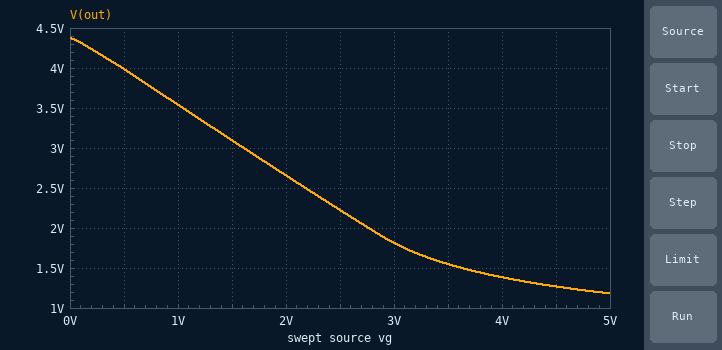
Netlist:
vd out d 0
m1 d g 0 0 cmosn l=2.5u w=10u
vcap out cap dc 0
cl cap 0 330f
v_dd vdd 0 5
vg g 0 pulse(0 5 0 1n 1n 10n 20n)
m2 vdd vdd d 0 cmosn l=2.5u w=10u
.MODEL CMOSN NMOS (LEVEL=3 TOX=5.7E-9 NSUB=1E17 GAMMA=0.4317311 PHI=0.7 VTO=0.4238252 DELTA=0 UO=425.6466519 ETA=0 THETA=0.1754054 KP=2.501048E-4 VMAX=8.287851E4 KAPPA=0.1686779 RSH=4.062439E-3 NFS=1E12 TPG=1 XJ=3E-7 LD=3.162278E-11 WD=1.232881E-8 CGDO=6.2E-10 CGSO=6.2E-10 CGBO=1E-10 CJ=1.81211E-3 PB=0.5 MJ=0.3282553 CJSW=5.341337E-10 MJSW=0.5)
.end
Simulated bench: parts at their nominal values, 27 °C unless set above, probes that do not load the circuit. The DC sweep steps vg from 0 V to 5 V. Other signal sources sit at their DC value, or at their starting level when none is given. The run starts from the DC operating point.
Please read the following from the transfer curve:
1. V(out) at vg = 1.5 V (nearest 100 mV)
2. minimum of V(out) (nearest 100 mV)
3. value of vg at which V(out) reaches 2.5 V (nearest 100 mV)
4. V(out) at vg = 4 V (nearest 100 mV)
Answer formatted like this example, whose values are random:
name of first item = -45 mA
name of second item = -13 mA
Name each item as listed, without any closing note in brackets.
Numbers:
V(out) at vg = 1.5 V = 3.1 V
minimum of V(out) = 1.2 V
value of vg at which V(out) reaches 2.5 V = 2.2 V
V(out) at vg = 4 V = 1.4 V
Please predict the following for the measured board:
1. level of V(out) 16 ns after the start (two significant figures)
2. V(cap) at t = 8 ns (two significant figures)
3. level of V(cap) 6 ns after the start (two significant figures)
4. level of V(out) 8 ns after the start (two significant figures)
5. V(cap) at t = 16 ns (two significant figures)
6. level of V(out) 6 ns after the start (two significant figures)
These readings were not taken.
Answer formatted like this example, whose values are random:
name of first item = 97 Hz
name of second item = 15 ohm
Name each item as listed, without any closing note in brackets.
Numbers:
level of V(out) 16 ns after the start = 3.9 V
V(cap) at t = 8 ns = 1.2 V
level of V(cap) 6 ns after the start = 1.2 V
level of V(out) 8 ns after the start = 1.2 V
V(cap) at t = 16 ns = 3.9 V
level of V(out) 6 ns after the start = 1.2 V
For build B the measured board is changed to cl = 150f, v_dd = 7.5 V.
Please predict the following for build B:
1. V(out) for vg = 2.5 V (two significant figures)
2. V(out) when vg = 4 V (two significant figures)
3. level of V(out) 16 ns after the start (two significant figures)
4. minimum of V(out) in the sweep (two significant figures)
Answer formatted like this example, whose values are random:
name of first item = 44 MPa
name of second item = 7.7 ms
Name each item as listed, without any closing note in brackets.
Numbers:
V(out) for vg = 2.5 V = 4.5 V
V(out) when vg = 4 V = 3.2 V
level of V(out) 16 ns after the start = 6.3 V
minimum of V(out) in the sweep = 2.5 V
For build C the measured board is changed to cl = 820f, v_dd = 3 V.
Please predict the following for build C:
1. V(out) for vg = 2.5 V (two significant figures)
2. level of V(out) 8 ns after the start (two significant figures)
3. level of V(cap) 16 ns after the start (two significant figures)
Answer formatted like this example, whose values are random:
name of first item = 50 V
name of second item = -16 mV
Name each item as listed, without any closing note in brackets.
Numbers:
V(out) for vg = 2.5 V = 760 mV
level of V(out) 8 ns after the start = 480 mV
level of V(cap) 16 ns after the start = 1.9 V
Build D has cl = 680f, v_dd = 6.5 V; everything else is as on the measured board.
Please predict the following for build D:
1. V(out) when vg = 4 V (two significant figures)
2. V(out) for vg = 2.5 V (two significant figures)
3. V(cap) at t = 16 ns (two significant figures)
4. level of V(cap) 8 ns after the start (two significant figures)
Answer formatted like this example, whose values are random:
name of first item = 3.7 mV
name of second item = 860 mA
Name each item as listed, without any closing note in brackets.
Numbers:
V(out) when vg = 4 V = 2.3 V
V(out) for vg = 2.5 V = 3.6 V
V(cap) at t = 16 ns = 5.1 V
level of V(cap) 8 ns after the start = 1.9 V
